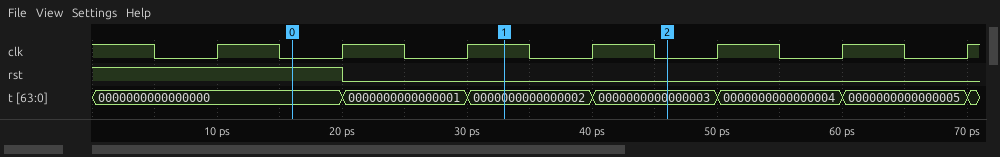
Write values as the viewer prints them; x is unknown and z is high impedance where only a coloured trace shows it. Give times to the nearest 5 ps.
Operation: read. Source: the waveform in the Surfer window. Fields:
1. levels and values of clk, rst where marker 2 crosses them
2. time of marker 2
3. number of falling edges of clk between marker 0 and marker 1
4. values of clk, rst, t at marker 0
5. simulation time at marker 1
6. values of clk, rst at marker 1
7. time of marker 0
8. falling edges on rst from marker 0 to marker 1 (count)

clk=0, rst=0
45 ps
1
clk=0, rst=1, t=0000000000000000
35 ps
clk=1, rst=0
15 ps
1
